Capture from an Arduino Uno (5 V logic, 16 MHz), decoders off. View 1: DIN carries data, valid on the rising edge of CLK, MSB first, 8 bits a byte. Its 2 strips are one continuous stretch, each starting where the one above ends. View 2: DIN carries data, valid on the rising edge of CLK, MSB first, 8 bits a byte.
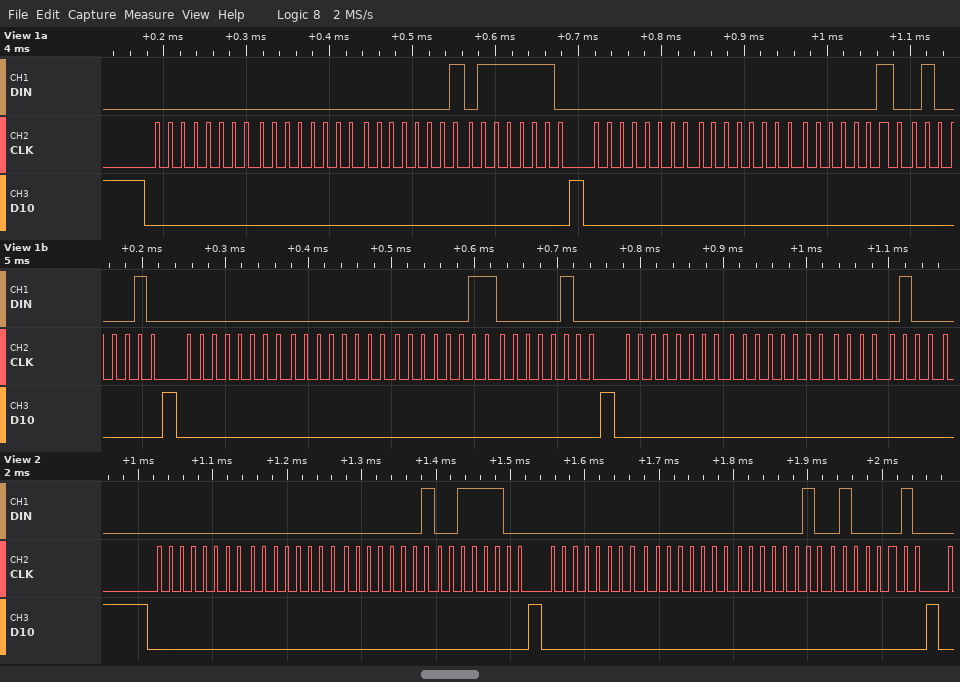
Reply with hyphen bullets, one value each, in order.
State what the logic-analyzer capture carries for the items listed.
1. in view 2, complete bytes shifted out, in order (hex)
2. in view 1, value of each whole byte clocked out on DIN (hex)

- 00 00 01 3C 00 00 02 42
- 00 00 01 7E 00 00 02 42 00 00 03 04 00 00 04
